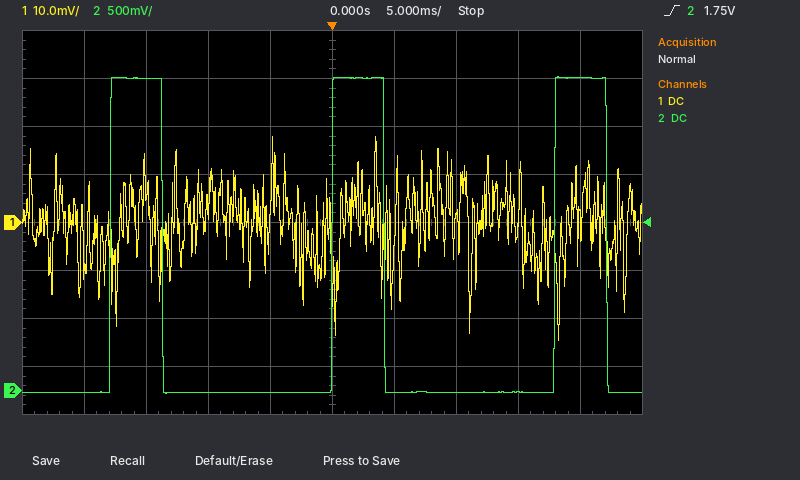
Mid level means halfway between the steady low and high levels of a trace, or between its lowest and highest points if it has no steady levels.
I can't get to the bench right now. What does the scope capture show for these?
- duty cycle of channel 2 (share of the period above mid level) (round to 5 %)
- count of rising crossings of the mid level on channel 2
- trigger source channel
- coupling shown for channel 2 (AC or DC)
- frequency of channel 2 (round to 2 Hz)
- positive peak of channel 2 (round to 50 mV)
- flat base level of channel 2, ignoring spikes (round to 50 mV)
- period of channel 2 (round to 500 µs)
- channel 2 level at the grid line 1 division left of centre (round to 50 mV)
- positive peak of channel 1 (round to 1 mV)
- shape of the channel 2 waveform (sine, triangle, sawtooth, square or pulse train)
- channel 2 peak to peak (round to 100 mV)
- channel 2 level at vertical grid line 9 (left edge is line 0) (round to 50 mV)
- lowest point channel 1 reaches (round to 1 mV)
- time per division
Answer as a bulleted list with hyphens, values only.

- 25 %
- 3
- channel 2
- DC
- 56 Hz
- 3.25 V
- 0 mV
- 18.0 ms
- 0 mV
- 18 mV
- pulse train
- 3.30 V
- 3.25 V
- -25 mV
- 5 ms
